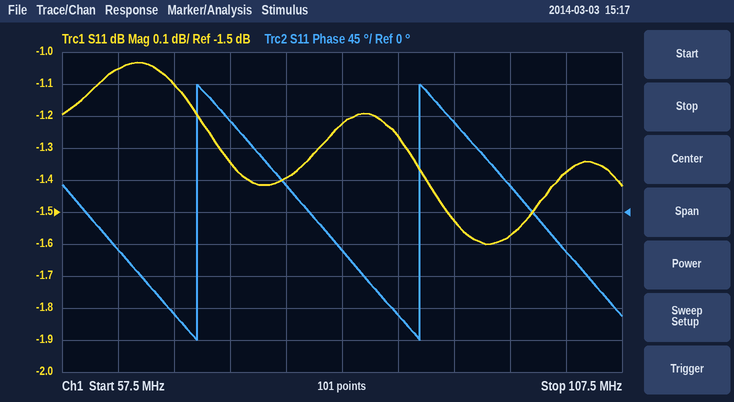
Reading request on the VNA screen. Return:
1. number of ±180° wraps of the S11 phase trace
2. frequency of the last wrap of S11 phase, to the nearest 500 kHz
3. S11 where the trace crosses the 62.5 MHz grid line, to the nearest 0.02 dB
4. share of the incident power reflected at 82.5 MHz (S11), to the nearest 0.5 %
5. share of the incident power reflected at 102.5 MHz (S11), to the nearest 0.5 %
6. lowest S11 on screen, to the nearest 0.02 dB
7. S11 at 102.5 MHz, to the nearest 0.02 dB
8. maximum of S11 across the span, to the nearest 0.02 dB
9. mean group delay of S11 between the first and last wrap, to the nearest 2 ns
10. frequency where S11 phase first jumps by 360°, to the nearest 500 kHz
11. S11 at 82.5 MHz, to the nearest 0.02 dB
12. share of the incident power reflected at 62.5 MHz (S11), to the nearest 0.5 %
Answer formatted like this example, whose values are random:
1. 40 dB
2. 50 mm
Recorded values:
1. 2
2. 89.5 MHz
3. -1.06 dB
4. 75.5 %
5. 73.0 %
6. -1.60 dB
7. -1.38 dB
8. -1.04 dB
9. 50 ns
10. 69.5 MHz
11. -1.22 dB
12. 78.5 %
